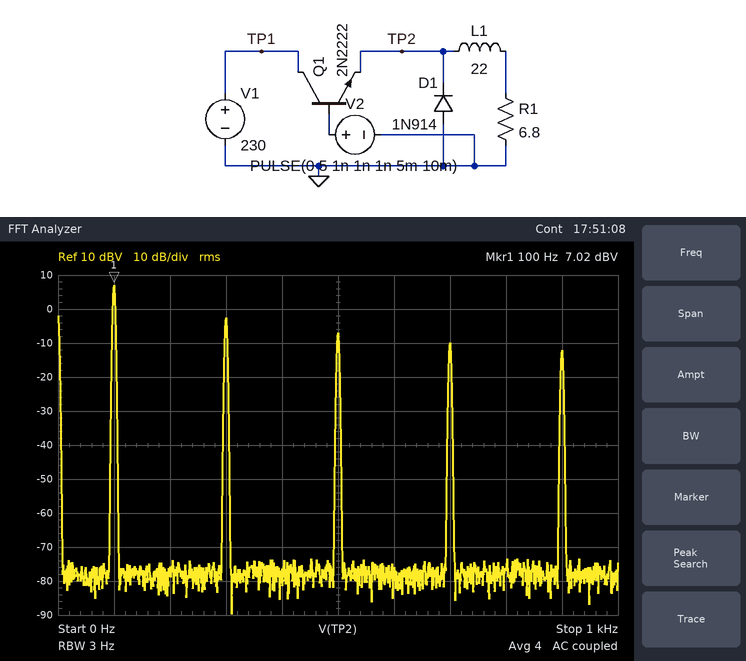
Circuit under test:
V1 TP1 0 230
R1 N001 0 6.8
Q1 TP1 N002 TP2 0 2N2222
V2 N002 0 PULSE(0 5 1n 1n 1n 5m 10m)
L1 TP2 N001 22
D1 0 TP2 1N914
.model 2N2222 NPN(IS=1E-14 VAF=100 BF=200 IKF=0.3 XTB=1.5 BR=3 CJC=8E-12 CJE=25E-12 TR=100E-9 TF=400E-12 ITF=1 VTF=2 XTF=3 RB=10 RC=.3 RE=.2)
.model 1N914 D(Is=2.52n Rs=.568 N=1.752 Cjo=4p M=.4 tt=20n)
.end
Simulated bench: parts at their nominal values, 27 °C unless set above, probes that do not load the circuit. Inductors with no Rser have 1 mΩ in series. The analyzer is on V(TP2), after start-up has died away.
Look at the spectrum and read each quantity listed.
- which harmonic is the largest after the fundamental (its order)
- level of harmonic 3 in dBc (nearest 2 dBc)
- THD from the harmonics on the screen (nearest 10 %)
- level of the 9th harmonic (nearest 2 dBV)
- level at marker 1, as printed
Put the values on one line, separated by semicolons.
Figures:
3; -10 dBc; 40 %; -12 dBV; 7.02 dBV
